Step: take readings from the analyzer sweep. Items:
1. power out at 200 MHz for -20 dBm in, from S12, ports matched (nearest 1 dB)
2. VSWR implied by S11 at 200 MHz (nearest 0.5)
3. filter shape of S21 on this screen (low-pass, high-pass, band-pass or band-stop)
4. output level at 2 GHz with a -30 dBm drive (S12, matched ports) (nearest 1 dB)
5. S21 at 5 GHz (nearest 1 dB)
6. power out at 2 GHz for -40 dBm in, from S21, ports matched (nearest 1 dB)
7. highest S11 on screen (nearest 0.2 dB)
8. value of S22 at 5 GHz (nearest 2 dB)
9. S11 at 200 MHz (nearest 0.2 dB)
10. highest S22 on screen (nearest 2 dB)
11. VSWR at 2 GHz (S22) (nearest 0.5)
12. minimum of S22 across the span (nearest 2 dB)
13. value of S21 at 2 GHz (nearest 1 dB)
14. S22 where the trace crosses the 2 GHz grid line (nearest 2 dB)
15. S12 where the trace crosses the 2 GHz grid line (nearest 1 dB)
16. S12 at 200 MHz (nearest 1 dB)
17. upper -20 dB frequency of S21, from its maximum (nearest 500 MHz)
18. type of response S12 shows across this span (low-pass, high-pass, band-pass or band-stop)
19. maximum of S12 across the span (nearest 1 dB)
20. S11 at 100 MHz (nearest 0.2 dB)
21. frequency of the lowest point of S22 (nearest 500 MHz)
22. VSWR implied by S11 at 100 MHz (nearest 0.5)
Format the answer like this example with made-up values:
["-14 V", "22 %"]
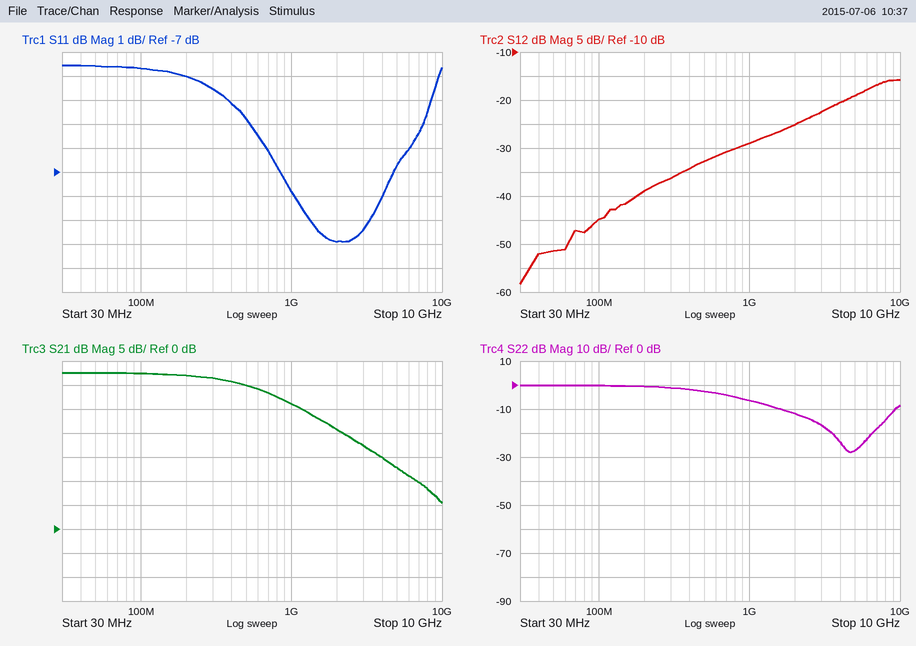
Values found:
["-59 dBm", "6.0", "low-pass", "-55 dBm", "13 dB", "-19 dBm", "-2.6 dB", "-28 dB", "-3.0 dB", "0 dB", "1.5", "-28 dB", "21 dB", "-12 dB", "-25 dB", "-39 dB", "5.0 GHz", "high-pass", "-16 dB", "-2.6 dB", "4.5 GHz", "6.5"]
